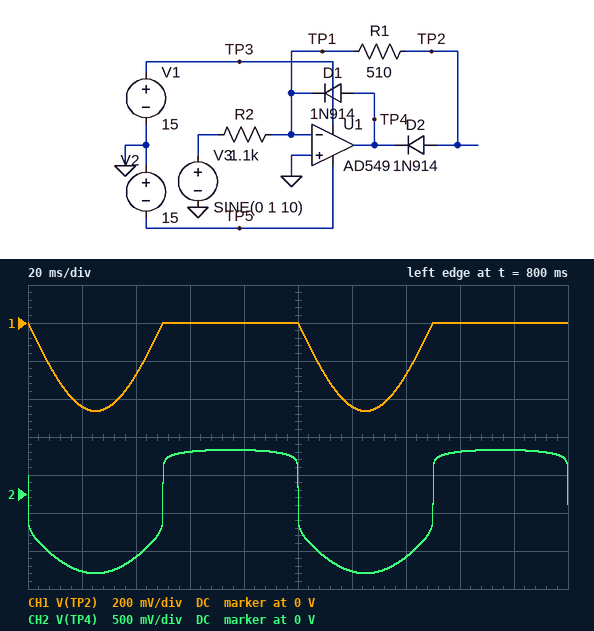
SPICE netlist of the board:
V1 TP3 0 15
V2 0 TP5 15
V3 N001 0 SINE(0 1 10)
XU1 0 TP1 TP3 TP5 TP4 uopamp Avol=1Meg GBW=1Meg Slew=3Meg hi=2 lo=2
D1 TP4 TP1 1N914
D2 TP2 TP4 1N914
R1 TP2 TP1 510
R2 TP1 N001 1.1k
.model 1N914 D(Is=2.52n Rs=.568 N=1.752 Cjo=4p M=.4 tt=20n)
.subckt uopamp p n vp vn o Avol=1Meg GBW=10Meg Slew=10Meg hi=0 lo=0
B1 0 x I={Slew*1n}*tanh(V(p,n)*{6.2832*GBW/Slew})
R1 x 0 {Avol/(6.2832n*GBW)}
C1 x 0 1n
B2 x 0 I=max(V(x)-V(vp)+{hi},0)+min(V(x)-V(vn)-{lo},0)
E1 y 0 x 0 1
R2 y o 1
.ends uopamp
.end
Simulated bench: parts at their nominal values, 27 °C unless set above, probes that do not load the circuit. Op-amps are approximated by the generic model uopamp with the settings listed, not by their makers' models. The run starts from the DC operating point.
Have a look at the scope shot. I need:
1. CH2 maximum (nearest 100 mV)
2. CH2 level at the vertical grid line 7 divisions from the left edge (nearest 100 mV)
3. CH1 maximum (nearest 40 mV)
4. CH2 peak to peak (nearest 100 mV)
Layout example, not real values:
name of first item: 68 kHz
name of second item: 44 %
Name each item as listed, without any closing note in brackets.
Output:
CH2 maximum: 600 mV
CH2 level at the vertical grid line 7 divisions from the left edge: -800 mV
CH1 maximum: 0 V
CH2 peak to peak: 1.6 V
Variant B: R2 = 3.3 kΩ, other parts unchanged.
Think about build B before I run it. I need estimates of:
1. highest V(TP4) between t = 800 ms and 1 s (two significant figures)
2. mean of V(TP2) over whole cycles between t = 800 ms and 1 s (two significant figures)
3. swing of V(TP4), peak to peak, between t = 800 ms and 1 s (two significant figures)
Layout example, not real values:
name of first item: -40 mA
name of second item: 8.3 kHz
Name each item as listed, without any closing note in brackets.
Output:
highest V(TP4) between t = 800 ms and 1 s: 530 mV
mean of V(TP2) over whole cycles between t = 800 ms and 1 s: -49 mV
swing of V(TP4), peak to peak, between t = 800 ms and 1 s: 1.2 V
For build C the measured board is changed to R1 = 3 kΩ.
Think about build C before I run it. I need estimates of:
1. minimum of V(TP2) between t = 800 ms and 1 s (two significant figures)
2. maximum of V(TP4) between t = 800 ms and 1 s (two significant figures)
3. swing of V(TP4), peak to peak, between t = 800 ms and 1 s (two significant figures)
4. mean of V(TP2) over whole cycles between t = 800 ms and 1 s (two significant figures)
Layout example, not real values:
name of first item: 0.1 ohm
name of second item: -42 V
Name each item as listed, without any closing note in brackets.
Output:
minimum of V(TP2) between t = 800 ms and 1 s: -2.7 V
maximum of V(TP4) between t = 800 ms and 1 s: 580 mV
swing of V(TP4), peak to peak, between t = 800 ms and 1 s: 3.9 V
mean of V(TP2) over whole cycles between t = 800 ms and 1 s: -870 mV
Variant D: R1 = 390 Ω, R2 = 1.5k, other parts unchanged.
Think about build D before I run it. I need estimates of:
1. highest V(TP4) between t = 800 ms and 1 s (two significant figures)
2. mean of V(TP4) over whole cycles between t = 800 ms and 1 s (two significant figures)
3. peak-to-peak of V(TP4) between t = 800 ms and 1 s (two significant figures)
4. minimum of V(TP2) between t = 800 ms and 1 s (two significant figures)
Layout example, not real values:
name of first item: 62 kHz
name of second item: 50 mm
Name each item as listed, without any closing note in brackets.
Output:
highest V(TP4) between t = 800 ms and 1 s: 570 mV
mean of V(TP4) over whole cycles between t = 800 ms and 1 s: -83 mV
peak-to-peak of V(TP4) between t = 800 ms and 1 s: 1.4 V
minimum of V(TP2) between t = 800 ms and 1 s: -260 mV
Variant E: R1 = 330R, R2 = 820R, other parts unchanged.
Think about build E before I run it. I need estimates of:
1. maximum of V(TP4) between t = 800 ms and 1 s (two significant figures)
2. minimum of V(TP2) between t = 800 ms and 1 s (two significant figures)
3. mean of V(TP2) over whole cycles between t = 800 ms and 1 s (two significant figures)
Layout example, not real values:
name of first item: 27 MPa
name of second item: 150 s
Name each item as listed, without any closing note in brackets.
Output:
maximum of V(TP4) between t = 800 ms and 1 s: 590 mV
minimum of V(TP2) between t = 800 ms and 1 s: -400 mV
mean of V(TP2) over whole cycles between t = 800 ms and 1 s: -130 mV
